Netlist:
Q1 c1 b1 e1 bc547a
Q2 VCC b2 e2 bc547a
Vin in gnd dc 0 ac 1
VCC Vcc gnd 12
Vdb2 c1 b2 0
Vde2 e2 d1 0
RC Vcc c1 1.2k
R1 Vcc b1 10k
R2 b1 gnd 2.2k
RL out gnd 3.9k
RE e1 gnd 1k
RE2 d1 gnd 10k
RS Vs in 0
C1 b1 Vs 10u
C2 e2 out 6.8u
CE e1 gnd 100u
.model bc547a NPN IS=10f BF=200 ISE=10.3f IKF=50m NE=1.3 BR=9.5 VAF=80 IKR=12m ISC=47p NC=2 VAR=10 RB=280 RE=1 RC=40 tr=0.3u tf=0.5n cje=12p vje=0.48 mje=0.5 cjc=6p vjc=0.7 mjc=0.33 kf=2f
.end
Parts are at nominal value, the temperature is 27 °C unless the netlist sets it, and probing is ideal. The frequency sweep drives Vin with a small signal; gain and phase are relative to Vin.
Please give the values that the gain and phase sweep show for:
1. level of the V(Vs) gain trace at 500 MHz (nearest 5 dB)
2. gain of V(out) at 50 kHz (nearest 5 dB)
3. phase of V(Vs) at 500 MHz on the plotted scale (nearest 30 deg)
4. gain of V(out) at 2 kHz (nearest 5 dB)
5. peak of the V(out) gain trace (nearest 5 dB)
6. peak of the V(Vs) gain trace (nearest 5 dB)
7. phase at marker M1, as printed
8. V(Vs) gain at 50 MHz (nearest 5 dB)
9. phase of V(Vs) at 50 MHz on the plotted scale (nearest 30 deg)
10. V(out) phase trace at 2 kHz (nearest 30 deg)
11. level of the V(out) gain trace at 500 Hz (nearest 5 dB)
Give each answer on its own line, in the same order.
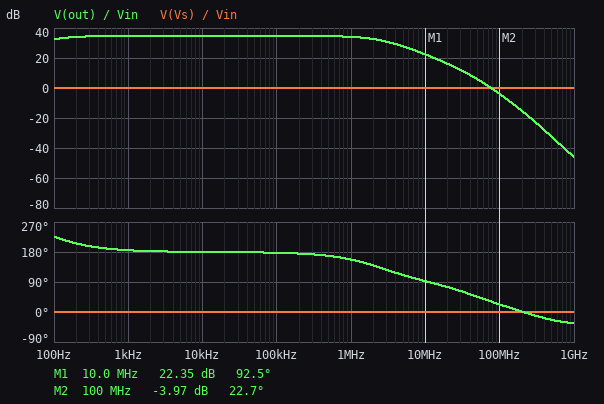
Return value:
0 dB
35 dB
0 deg
35 dB
35 dB
0 dB
92.5 deg
0 dB
0 deg
180 deg
35 dB
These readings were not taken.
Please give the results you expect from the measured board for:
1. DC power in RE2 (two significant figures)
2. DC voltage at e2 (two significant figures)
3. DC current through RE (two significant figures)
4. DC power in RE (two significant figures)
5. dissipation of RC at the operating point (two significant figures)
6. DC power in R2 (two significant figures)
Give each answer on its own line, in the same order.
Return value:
9.2 mW
9.6 V
1.5 mA
2.2 mW
2.6 mW
2.1 mW
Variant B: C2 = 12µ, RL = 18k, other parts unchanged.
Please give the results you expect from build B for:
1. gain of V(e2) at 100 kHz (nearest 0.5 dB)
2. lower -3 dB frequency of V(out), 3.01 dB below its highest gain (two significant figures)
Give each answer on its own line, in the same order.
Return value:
35.0 dB
82 Hz
